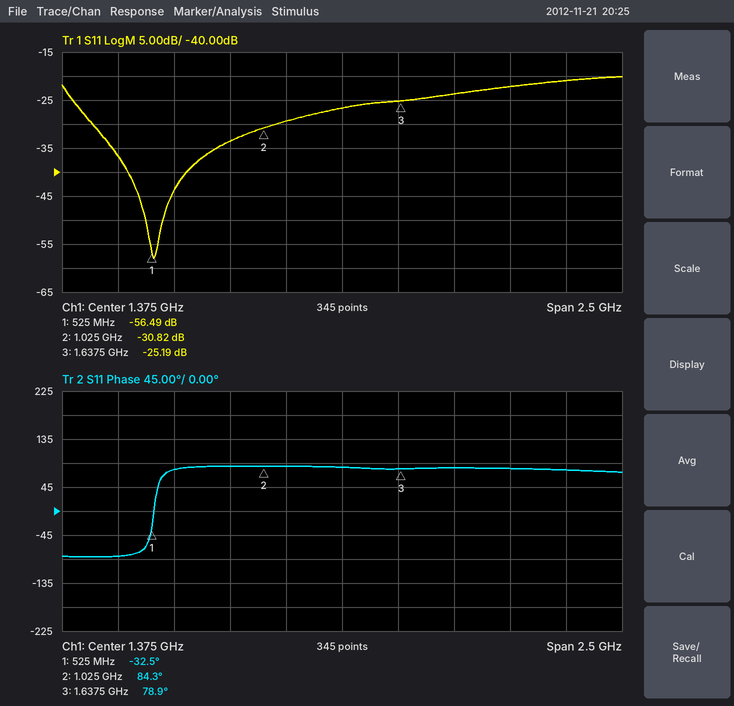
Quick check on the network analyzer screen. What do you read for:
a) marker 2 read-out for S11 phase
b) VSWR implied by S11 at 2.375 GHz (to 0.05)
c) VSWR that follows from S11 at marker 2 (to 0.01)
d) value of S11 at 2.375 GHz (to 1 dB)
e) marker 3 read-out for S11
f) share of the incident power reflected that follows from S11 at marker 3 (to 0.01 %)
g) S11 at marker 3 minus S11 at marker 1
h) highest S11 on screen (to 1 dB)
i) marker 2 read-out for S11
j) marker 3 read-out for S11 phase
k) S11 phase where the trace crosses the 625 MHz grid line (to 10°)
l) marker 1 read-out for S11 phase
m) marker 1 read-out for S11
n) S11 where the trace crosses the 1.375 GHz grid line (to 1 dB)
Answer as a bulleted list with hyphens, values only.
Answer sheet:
- 84.3°
- 1.20
- 1.06
- -21 dB
- -25.19 dB
- 0.30 %
- 31.30 dB
- -20 dB
- -30.82 dB
- 78.9°
- 80°
- -32.5°
- -56.49 dB
- -27 dB
